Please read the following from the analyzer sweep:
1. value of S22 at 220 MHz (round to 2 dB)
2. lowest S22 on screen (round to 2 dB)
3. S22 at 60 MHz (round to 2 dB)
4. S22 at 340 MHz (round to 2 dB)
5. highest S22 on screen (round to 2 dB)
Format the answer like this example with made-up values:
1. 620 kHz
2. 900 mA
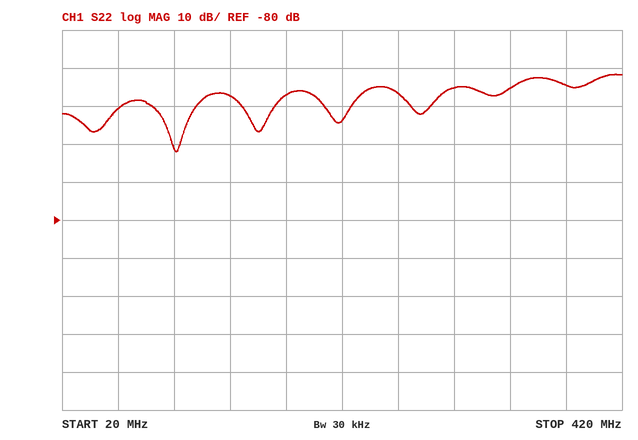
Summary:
1. -54 dB
2. -62 dB
3. -50 dB
4. -46 dB
5. -42 dB
